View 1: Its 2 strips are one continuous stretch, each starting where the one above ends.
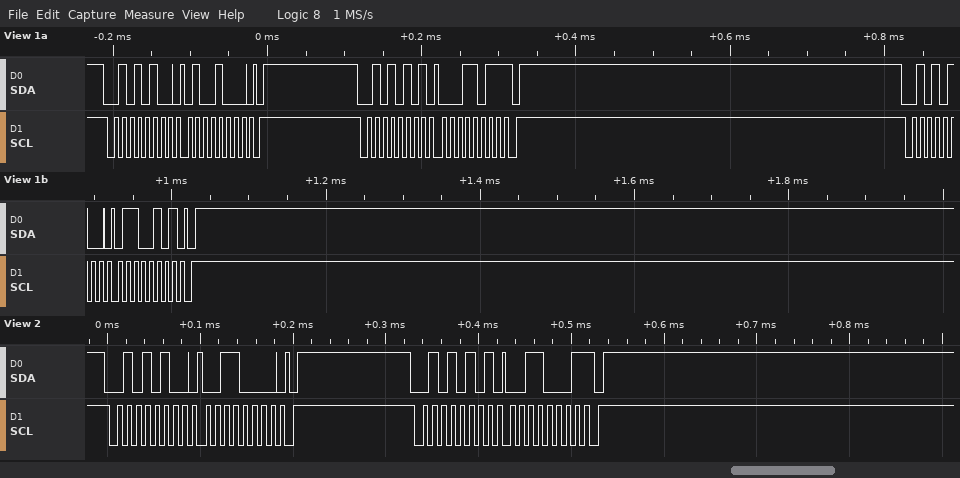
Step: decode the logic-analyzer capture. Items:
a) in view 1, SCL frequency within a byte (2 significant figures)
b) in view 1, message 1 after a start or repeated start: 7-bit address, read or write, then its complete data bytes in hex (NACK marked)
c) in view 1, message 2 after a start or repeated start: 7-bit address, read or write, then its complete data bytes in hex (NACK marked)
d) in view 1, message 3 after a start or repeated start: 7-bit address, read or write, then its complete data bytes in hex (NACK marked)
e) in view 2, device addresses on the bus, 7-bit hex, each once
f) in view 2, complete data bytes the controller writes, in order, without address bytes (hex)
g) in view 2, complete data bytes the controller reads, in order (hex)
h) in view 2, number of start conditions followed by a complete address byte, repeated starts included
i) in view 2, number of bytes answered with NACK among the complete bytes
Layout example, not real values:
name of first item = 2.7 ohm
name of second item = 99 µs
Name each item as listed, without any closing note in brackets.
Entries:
in view 1, SCL frequency within a byte = 100 kHz
in view 1, message 1 after a start or repeated start: 7-bit address, read or write, then its complete data bytes in hex = 0x2A write: 48
in view 1, message 2 after a start or repeated start: 7-bit address, read or write, then its complete data bytes in hex = 0x2A read: 1B NACK
in view 1, message 3 after a start or repeated start: 7-bit address, read or write, then its complete data bytes in hex = 0x2A write: 65
in view 2, device addresses on the bus, 7-bit hex, each once = 0x2A
in view 2, complete data bytes the controller writes, in order, without address bytes = 30
in view 2, complete data bytes the controller reads, in order = 31
in view 2, number of start conditions followed by a complete address byte, repeated starts included = 2
in view 2, number of bytes answered with NACK among the complete bytes = 1
